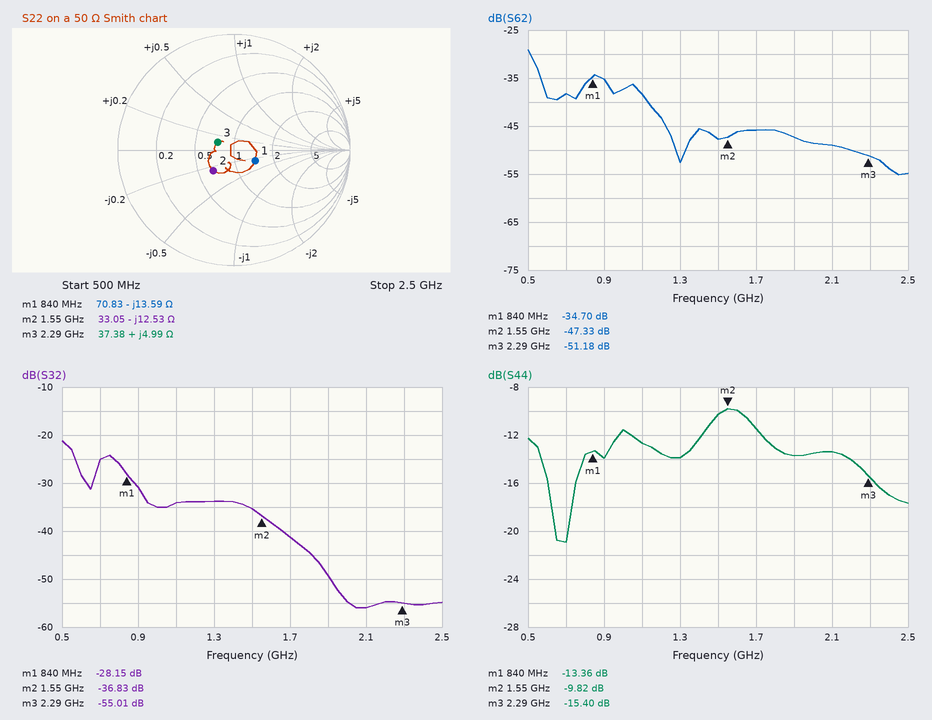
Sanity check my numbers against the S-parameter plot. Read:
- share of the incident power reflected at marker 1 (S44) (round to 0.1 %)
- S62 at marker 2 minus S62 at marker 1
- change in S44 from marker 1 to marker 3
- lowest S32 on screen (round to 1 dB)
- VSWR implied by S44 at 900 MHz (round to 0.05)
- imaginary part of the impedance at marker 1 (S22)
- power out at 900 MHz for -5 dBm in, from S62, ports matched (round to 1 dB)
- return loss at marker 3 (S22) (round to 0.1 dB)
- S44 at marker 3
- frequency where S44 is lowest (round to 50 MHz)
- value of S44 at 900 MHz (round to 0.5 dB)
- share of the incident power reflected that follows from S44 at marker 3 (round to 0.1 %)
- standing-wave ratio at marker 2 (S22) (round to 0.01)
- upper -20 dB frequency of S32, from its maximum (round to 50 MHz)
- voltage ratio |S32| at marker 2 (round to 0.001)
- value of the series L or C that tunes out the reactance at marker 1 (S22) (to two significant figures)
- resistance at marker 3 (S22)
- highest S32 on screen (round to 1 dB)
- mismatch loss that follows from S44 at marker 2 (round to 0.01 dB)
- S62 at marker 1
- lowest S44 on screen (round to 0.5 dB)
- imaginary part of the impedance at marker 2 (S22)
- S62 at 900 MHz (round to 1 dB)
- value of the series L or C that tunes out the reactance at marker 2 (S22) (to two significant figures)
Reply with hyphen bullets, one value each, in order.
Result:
- 4.6 %
- -12.63 dB
- -2.04 dB
- -56 dB
- 1.50
- -13.59 Ω
- -40 dBm
- 16.2 dB
- -15.40 dB
- 700 MHz
- -14.0 dB
- 2.9 %
- 1.67
- 1.70 GHz
- 0.014
- 2.6 nH
- 37.38 Ω
- -21 dB
- 0.48 dB
- -34.70 dB
- -21.0 dB
- -12.53 Ω
- -35 dB
- 1.3 nH
